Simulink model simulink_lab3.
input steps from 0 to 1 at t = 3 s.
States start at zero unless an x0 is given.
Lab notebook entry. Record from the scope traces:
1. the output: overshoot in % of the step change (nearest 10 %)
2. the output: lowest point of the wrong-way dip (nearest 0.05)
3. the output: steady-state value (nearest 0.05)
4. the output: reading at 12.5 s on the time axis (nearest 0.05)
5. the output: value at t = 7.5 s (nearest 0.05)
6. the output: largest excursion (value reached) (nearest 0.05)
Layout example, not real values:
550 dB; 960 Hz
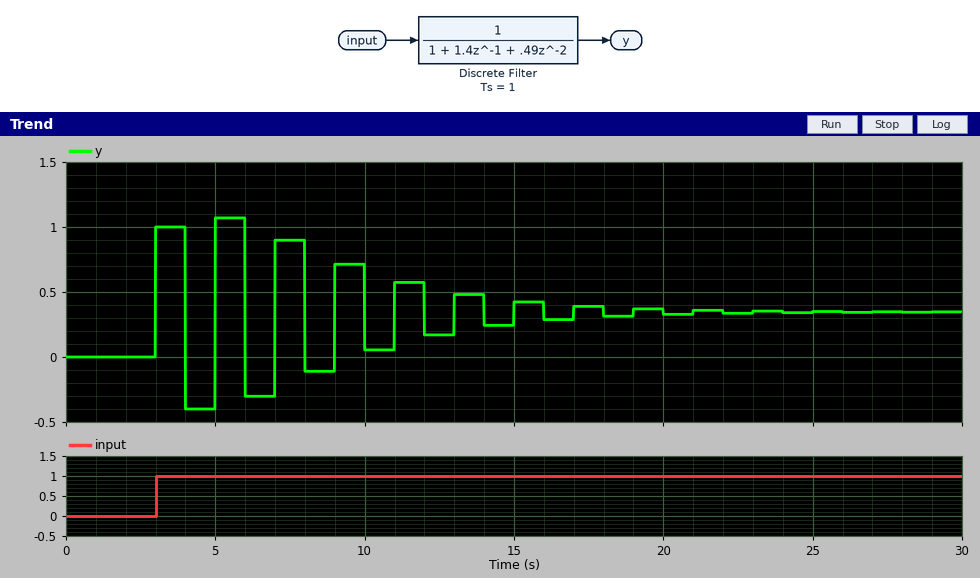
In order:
210 %; -0.40; 0.35; 0.15; 0.90; 1.05
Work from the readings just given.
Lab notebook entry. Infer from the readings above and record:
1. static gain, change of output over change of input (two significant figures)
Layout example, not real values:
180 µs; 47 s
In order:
0.35
